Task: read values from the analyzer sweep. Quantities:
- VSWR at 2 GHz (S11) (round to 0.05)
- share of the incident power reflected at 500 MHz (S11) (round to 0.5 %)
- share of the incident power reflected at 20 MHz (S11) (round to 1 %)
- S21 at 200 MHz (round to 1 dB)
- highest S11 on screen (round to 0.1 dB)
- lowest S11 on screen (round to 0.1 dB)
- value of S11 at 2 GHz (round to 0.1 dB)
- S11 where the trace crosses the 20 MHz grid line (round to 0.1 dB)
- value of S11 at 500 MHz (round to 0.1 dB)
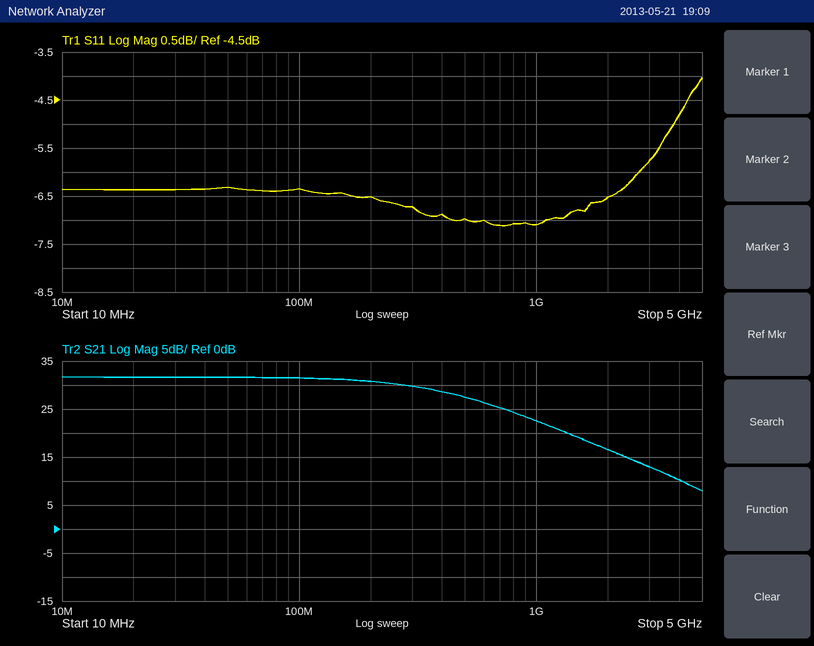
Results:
2.80
20.0 %
23 %
31 dB
-4.0 dB
-7.1 dB
-6.5 dB
-6.4 dB
-7.0 dB
